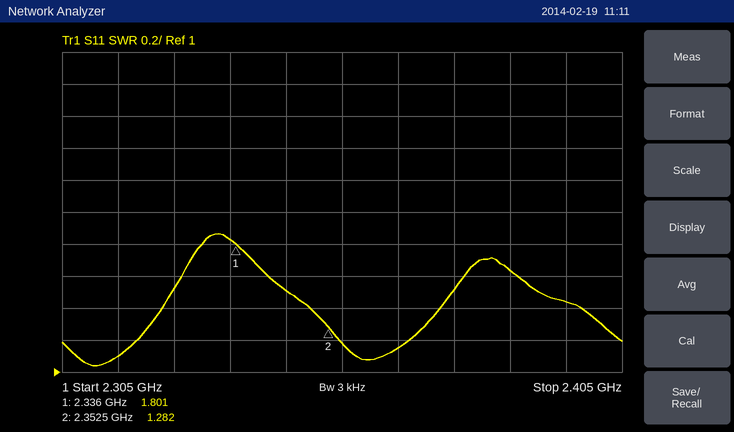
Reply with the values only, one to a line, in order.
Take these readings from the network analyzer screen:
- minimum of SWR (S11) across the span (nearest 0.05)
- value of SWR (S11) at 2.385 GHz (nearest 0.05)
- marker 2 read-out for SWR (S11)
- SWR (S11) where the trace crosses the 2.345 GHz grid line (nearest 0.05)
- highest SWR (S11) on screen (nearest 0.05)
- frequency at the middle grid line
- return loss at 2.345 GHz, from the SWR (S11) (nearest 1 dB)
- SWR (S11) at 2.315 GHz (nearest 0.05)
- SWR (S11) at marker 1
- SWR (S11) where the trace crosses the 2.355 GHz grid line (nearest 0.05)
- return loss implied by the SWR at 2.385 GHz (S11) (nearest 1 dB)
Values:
1.05
1.65
1.282
1.50
1.85
2.355 GHz
14 dB
1.10
1.801
1.20
12 dB
